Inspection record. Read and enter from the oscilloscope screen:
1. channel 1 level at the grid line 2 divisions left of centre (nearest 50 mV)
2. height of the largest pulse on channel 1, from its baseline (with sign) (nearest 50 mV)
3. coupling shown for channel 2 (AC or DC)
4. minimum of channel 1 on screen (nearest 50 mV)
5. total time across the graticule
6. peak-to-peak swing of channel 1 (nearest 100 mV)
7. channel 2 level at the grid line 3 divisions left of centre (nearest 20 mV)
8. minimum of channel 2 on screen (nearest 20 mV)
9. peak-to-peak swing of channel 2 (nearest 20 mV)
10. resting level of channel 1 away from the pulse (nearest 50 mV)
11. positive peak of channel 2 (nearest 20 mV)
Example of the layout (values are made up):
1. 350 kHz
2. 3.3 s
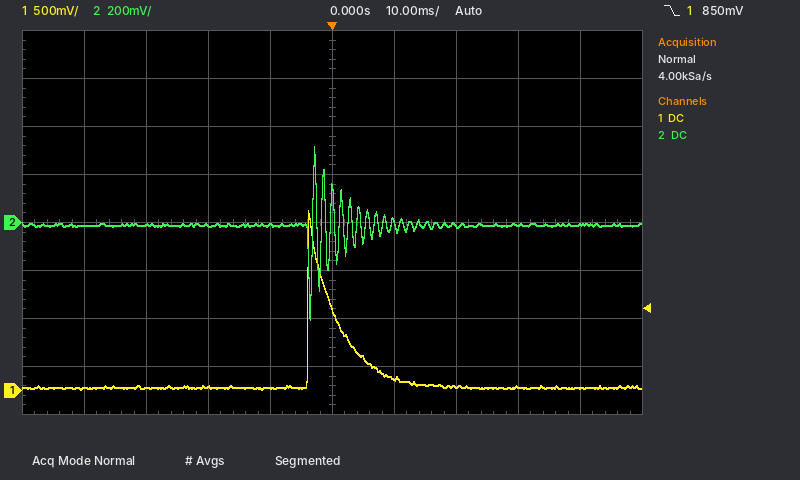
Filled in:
1. 50 mV
2. +1.85 V
3. DC
4. 0 mV
5. 100 ms
6. 1.90 V
7. 0 mV
8. -400 mV
9. 720 mV
10. 50 mV
11. 320 mV
